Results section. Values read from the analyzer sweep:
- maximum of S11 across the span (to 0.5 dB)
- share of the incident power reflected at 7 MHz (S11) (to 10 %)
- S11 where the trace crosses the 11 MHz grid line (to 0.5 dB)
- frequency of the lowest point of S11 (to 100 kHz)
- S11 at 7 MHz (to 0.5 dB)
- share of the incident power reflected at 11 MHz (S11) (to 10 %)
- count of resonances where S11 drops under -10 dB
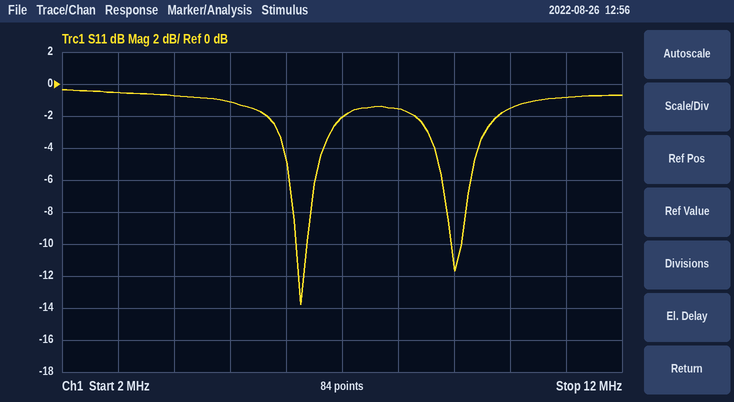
-0.5 dB
60 %
-1.0 dB
6.3 MHz
-2.0 dB
80 %
2
